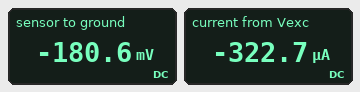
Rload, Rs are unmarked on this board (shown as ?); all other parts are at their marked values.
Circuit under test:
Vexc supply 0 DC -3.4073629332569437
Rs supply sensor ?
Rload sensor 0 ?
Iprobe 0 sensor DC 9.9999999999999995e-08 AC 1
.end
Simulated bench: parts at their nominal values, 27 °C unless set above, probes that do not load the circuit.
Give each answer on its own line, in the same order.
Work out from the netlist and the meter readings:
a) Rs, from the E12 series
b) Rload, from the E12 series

10 kΩ
560 Ω
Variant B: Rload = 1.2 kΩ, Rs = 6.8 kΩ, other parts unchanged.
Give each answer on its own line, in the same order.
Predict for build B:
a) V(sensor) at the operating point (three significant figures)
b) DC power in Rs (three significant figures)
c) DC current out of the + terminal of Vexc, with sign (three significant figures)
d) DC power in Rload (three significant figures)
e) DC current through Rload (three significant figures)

-511 mV
1.23 mW
-426 µA
218 µW
426 µA
